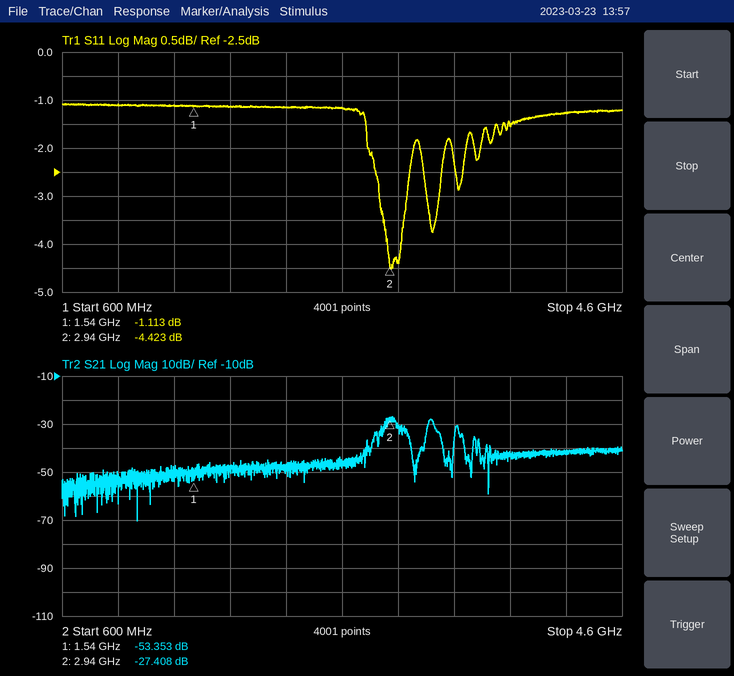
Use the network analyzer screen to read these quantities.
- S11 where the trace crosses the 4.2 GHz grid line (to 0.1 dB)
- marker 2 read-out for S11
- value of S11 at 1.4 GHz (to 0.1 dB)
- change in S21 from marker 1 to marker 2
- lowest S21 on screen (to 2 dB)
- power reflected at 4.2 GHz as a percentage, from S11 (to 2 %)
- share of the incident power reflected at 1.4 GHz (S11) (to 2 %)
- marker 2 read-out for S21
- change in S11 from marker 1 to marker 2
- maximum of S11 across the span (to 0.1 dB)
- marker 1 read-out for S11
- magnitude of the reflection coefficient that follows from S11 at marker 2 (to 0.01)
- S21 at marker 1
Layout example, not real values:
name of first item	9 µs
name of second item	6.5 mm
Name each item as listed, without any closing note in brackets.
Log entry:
S11 where the trace crosses the 4.2 GHz grid line	-1.3 dB
marker 2 read-out for S11	-4.423 dB
value of S11 at 1.4 GHz	-1.1 dB
change in S21 from marker 1 to marker 2	25.945 dB
lowest S21 on screen	-70 dB
power reflected at 4.2 GHz as a percentage, from S11	74 %
share of the incident power reflected at 1.4 GHz (S11)	78 %
marker 2 read-out for S21	-27.408 dB
change in S11 from marker 1 to marker 2	-3.310 dB
maximum of S11 across the span	-1.1 dB
marker 1 read-out for S11	-1.113 dB
magnitude of the reflection coefficient that follows from S11 at marker 2	0.60
S21 at marker 1	-53.353 dB
